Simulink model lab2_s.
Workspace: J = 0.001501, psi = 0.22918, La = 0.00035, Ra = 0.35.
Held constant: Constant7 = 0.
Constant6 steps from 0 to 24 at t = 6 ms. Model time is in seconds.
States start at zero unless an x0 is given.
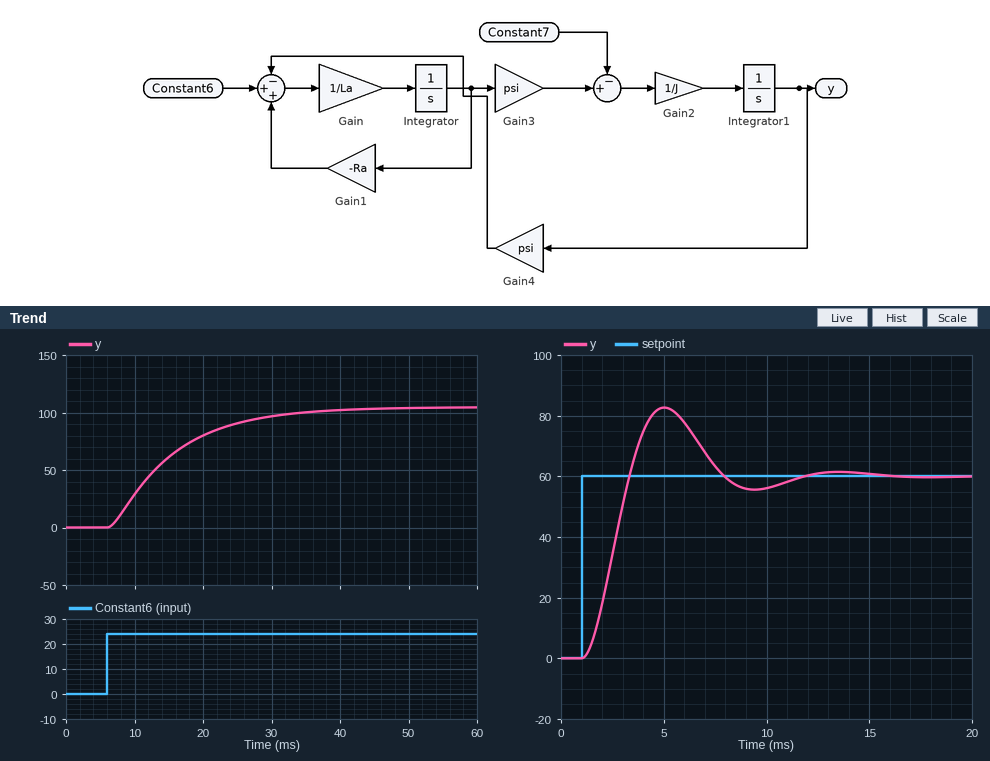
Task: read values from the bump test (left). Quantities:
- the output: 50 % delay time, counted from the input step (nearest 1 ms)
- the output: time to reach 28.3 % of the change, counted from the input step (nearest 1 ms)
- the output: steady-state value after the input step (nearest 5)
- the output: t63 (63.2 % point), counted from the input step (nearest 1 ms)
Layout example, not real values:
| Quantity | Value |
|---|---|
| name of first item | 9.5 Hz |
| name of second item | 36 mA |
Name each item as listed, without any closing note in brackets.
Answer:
| Quantity | Value |
|---|---|
| the output: 50 % delay time, counted from the input step | 7 ms |
| the output: time to reach 28.3 % of the change, counted from the input step | 4 ms |
| the output: steady-state value after the input step | 105 |
| the output: t63 (63.2 % point), counted from the input step | 10 ms |
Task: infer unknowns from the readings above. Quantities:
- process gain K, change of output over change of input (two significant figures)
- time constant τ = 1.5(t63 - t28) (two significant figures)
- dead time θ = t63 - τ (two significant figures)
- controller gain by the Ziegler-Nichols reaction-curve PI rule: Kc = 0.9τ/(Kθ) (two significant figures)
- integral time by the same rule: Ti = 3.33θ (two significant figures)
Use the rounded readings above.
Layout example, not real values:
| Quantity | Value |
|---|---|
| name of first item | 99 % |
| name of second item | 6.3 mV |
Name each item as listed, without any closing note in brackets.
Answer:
| Quantity | Value |
|---|---|
| process gain K, change of output over change of input | 4.4 |
| time constant τ = 1.5(t63 - t28) | 9.0 ms |
| dead time θ = t63 - τ | 1.0 ms |
| controller gain by the Ziegler-Nichols reaction-curve PI rule: Kc = 0.9τ/(Kθ) | 1.8 |
| integral time by the same rule: Ti = 3.33θ | 3.3 ms |
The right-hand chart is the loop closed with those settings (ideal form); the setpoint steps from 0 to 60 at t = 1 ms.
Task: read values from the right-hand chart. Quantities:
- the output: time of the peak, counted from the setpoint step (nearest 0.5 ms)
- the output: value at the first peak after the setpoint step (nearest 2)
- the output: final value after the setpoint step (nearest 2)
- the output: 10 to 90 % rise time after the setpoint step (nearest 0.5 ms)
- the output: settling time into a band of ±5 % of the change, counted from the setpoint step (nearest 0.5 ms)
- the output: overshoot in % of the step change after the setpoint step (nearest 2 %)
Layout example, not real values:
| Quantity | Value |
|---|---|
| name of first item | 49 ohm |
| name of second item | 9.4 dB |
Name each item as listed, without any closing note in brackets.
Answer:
| Quantity | Value |
|---|---|
| the output: time of the peak, counted from the setpoint step | 4.0 ms |
| the output: value at the first peak after the setpoint step | 82 |
| the output: final value after the setpoint step | 60 |
| the output: 10 to 90 % rise time after the setpoint step | 1.5 ms |
| the output: settling time into a band of ±5 % of the change, counted from the setpoint step | 9.5 ms |
| the output: overshoot in % of the step change after the setpoint step | 38 % |
